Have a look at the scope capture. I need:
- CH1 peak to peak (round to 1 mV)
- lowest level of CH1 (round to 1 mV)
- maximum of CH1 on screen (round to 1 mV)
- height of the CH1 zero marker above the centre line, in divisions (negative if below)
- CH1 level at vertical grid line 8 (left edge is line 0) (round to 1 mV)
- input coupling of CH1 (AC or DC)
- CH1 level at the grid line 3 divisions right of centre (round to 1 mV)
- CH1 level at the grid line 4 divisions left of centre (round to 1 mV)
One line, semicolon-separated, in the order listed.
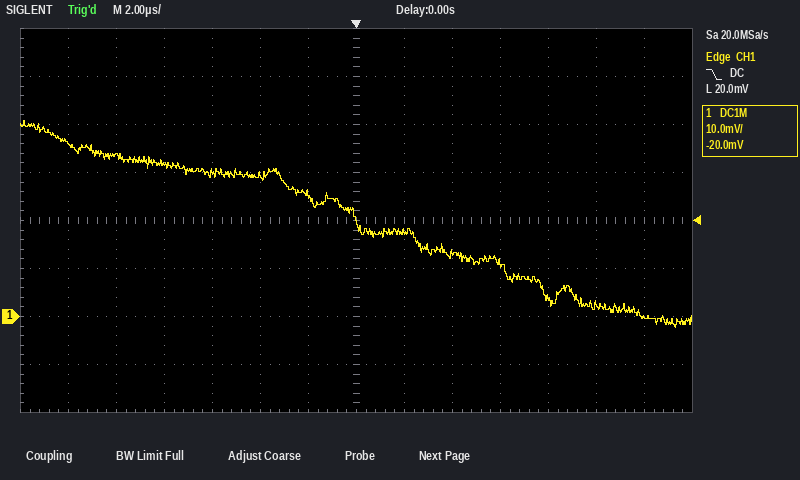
43 mV; -2 mV; 41 mV; -2.0 div; 18 mV; DC; 11 mV; 32 mV
